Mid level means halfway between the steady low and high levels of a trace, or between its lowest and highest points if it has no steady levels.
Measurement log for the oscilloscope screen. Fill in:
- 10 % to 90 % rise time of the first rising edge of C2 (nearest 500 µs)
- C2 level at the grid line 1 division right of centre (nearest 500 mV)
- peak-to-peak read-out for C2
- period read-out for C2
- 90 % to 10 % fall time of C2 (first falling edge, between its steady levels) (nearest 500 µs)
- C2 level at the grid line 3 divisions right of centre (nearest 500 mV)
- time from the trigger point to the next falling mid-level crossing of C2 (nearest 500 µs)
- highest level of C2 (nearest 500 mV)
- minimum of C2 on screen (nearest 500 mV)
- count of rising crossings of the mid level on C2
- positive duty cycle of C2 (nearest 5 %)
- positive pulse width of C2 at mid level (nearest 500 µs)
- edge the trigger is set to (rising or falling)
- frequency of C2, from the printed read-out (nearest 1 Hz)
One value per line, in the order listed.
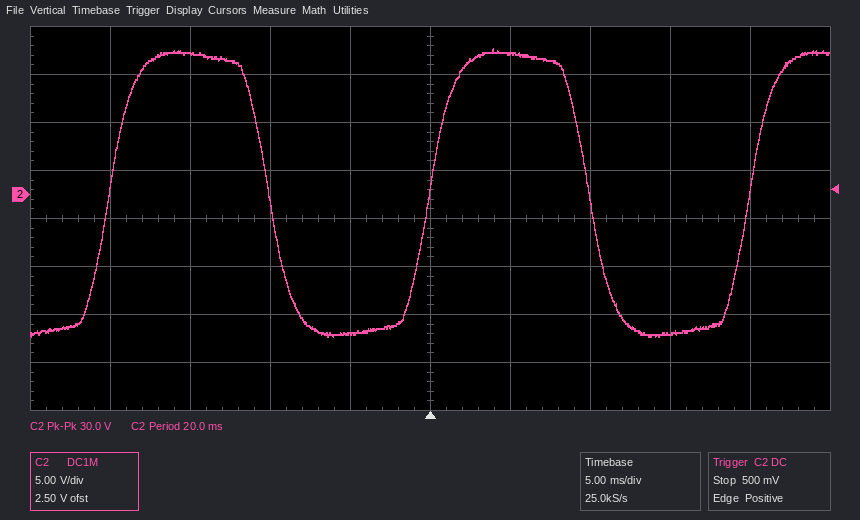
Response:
3.0 ms
14.5 V
30.0 V
20.0 ms
3.0 ms
-14.5 V
10.0 ms
15.0 V
-15.0 V
3
50 %
10.0 ms
rising
50 Hz
